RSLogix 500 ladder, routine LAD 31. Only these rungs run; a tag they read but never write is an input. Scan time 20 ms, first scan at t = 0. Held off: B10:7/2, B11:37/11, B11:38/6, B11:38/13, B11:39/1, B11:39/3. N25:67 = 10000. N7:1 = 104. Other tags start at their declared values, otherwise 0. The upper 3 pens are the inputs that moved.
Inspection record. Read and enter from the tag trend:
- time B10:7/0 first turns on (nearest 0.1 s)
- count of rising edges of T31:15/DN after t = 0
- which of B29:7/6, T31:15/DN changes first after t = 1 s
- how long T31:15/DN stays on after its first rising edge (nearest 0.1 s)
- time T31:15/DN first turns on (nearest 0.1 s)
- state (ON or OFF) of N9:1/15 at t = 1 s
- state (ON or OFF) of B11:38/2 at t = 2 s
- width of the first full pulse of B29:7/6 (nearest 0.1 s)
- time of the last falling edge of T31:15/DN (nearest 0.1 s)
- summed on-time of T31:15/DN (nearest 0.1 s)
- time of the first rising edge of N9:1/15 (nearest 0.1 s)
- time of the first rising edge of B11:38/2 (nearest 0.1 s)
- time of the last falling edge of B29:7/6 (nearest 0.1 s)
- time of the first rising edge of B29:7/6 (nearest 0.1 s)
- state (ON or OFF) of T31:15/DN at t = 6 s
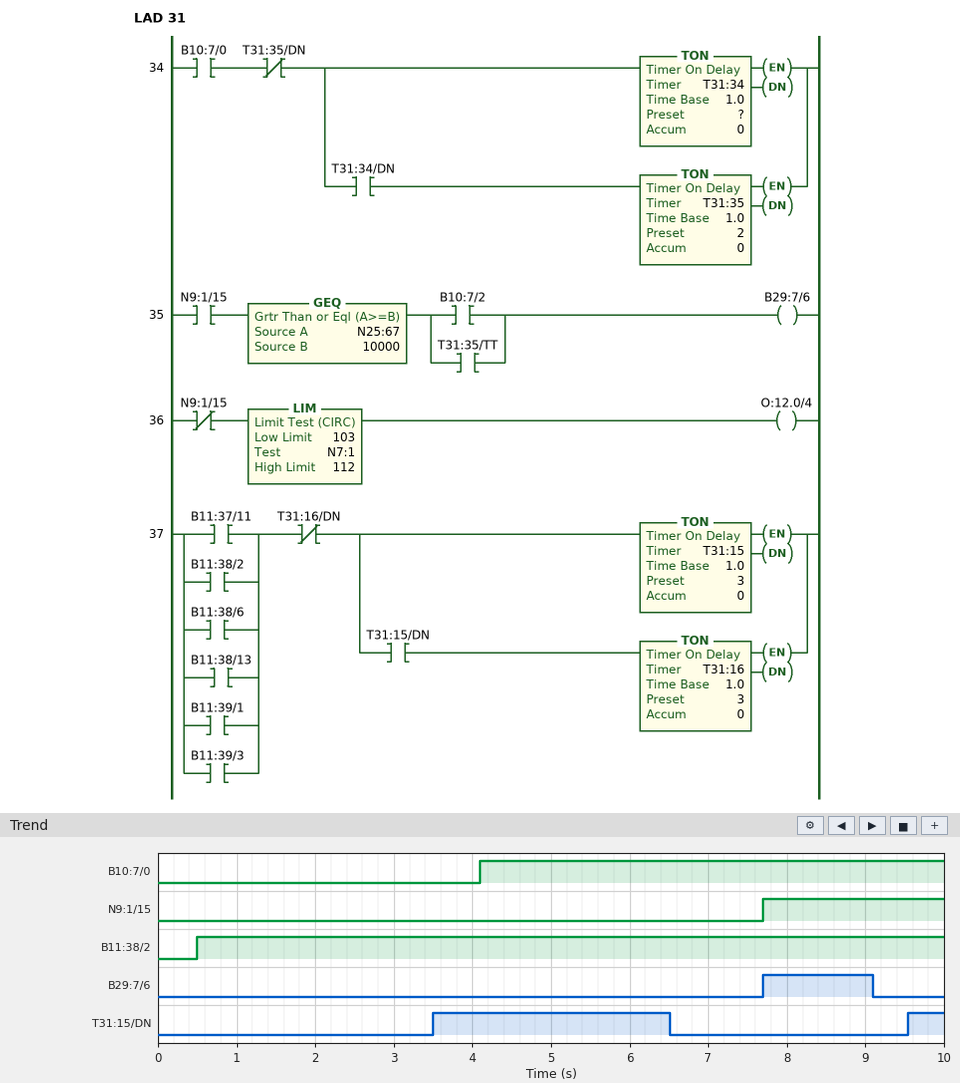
4.1 s
2
T31:15/DN
3.0 s
3.5 s
OFF
ON
1.4 s
6.5 s
3.5 s
7.7 s
0.5 s
9.1 s
7.7 s
ON
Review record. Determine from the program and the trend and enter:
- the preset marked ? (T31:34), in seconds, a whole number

3 s
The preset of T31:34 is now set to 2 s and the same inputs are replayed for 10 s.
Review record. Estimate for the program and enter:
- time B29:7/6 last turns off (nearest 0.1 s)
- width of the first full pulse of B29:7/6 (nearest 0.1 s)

8.1 s
0.4 s
